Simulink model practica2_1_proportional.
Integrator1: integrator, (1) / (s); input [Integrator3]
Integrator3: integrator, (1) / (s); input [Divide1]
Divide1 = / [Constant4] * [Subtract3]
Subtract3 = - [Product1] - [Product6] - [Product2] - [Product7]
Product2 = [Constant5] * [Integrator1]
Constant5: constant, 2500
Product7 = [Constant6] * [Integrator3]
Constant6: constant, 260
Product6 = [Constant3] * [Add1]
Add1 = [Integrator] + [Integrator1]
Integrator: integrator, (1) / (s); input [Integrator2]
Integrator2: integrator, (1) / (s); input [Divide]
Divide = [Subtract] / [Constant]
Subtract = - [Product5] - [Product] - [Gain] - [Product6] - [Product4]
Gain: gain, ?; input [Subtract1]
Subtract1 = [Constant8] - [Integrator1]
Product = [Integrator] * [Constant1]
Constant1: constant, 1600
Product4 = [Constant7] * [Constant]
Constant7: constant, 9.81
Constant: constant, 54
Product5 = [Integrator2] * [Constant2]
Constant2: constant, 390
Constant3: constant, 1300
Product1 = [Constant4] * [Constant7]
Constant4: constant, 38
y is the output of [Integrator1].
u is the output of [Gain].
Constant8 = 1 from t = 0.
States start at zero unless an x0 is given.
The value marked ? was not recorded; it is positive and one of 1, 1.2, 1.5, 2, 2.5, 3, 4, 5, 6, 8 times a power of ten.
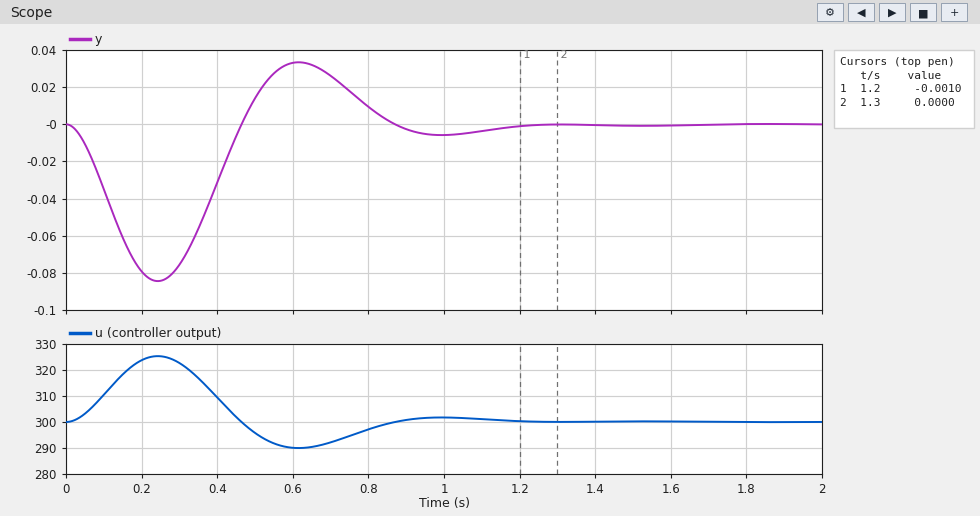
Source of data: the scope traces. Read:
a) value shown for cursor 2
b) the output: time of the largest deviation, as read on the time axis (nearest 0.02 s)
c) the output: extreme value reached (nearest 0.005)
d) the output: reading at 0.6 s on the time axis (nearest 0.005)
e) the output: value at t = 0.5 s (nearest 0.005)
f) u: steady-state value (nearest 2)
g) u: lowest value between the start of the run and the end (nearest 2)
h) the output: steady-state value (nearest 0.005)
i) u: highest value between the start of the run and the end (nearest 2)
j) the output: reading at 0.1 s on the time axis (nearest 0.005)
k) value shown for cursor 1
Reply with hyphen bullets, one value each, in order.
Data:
- 0.0000
- 0.24 s
- -0.085
- 0.035
- 0.015
- 300
- 290
- 0.000
- 326
- -0.035
- -0.0010
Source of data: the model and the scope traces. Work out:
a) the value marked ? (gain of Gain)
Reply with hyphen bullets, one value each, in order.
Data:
- 300
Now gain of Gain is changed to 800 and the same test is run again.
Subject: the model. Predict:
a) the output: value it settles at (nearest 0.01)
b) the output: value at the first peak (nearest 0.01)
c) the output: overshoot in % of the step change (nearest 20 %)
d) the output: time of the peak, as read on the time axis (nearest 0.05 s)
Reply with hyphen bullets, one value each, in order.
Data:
- 0.06
- 0.12
- 100 %
- 0.60 s
